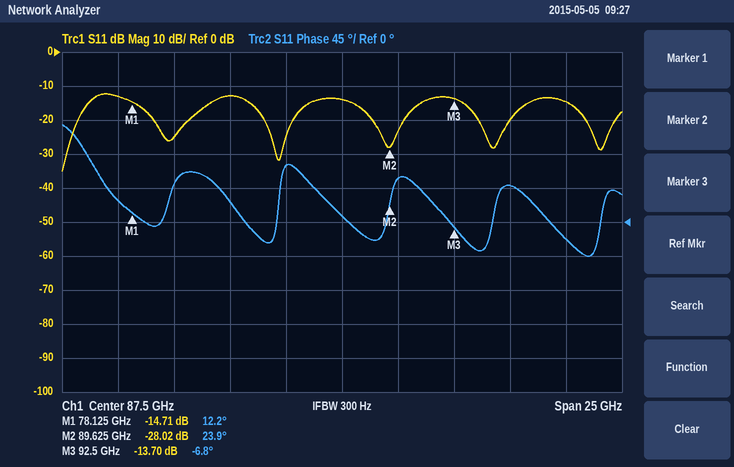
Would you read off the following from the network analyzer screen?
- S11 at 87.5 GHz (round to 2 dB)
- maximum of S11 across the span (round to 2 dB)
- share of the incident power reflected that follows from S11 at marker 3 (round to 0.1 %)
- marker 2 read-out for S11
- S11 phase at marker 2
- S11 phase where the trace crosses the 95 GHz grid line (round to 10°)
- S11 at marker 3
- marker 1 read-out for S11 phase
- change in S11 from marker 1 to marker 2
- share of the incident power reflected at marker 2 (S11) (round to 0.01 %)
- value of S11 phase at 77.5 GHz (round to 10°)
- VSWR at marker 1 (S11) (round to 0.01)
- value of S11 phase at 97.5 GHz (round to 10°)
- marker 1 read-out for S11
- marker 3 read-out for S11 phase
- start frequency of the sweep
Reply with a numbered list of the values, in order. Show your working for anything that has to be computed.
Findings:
1. -14 dB
2. -12 dB
3. 10^(-13.7/10) ≈ 4.3 %
4. -28.02 dB
5. 23.9°
6. 50°
7. -13.70 dB
8. 12.2°
9. -28.02 − (-14.71) = -13.31 dB
10. 10^(-28.02/10) ≈ 0.16 %
11. 30°
12. (1 + 0.1839)/(1 − 0.1839) ≈ 1.45
13. -20°
14. -14.71 dB
15. -6.8°
16. 75 GHz
